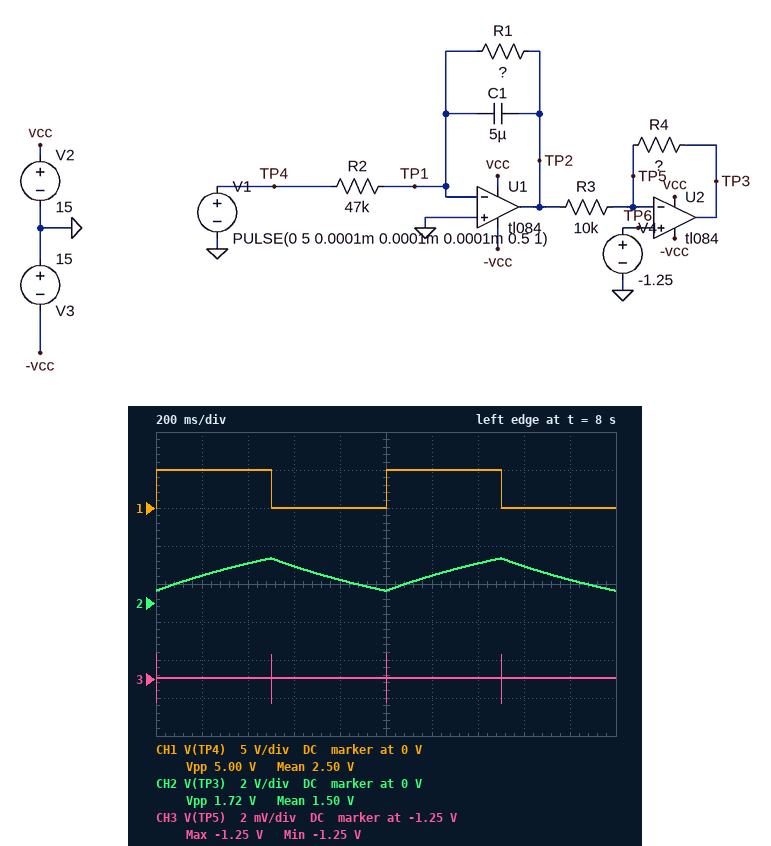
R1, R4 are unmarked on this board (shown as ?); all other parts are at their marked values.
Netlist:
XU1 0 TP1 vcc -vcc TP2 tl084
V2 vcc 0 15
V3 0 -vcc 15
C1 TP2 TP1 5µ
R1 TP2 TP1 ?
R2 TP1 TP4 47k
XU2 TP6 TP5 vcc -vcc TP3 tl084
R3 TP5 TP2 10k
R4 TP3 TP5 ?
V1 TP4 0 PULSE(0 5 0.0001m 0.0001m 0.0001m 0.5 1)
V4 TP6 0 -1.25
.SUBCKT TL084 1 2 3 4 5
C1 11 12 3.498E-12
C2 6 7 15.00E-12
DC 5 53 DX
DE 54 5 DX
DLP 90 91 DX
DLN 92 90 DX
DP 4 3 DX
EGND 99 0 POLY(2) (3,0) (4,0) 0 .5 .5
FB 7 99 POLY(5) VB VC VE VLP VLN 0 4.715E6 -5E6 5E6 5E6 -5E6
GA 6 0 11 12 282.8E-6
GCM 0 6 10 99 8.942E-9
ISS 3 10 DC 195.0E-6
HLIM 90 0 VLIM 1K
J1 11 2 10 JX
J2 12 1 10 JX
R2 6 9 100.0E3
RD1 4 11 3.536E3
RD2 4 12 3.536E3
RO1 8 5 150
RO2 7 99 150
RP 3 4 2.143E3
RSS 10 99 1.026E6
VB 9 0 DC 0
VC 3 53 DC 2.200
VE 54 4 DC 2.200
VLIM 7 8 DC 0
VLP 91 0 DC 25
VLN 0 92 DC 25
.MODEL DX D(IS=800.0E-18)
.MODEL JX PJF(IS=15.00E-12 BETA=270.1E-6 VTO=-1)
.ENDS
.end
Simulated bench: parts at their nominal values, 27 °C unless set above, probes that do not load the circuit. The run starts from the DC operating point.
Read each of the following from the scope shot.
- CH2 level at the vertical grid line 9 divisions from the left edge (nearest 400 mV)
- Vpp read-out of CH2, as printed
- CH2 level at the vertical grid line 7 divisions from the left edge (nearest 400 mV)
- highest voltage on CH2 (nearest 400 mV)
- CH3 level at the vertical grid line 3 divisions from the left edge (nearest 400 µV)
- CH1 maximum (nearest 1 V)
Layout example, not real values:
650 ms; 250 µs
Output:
1.2 V; 1.72 V; 2.0 V; 2.4 V; -1.2500 V; 5 V
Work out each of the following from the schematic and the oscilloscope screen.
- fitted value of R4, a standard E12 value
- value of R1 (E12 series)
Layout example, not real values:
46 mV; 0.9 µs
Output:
3.3 kΩ; 180 kΩ
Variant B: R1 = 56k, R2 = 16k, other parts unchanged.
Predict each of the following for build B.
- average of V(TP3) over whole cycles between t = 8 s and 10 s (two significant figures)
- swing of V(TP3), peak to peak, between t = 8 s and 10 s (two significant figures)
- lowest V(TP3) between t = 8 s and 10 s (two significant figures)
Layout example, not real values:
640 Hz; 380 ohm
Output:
1.1 V; 3.7 V; -880 mV
